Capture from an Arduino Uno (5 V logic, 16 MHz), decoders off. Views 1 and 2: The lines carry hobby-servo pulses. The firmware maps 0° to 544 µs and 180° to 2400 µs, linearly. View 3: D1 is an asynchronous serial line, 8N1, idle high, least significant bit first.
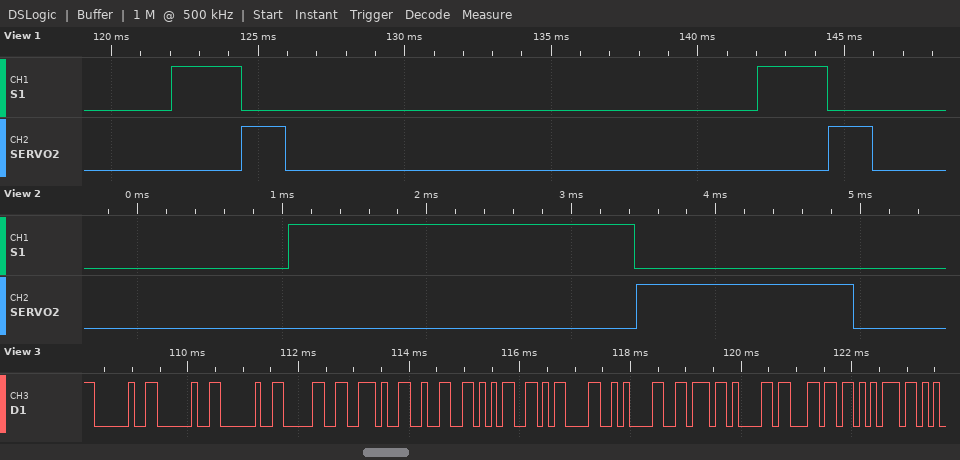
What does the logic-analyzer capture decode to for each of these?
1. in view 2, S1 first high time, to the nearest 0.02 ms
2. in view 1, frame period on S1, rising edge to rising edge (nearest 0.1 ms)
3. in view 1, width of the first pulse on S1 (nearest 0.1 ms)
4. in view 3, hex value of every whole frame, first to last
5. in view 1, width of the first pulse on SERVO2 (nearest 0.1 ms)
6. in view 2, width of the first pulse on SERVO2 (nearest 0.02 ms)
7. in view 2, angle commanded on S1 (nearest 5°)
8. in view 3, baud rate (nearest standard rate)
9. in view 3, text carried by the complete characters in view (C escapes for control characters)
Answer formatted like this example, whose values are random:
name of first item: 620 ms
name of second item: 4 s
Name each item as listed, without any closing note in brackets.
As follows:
in view 2, S1 first high time, to the nearest 0.02 ms: 2.40 ms
in view 1, frame period on S1, rising edge to rising edge: 20.0 ms
in view 1, width of the first pulse on S1: 2.4 ms
in view 3, hex value of every whole frame, first to last: 20 20 20 30 2E 32 35 0D 0A 76 61 6C 75
in view 1, width of the first pulse on SERVO2: 1.5 ms
in view 2, width of the first pulse on SERVO2: 1.50 ms
in view 2, angle commanded on S1: 180°
in view 3, baud rate: 9600 baud
in view 3, text carried by the complete characters in view: "   0.25\r\nvalu"
